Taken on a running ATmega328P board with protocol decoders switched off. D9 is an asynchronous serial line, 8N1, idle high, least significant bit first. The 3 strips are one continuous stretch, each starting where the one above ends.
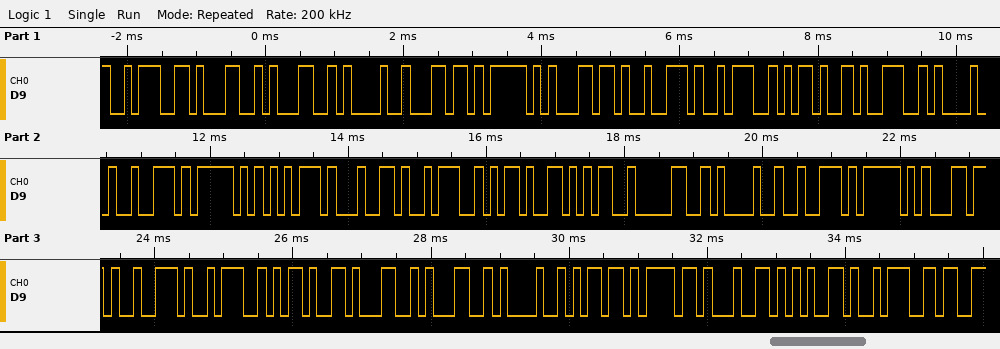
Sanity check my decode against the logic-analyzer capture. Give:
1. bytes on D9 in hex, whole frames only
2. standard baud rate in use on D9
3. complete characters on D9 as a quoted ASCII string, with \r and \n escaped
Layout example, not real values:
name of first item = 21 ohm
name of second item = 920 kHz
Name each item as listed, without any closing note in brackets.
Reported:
bytes on D9 in hex, whole frames only = 0x3A 0x31 0x31 0x21 0x6C 0x5F 0x6C 0x72 0x3A 0x2D 0x39 0x21 0x72 0x5F 0x75 0x64 0x3A 0x2D 0x35 0x30 0x21 0x72 0x5F 0x6C 0x72 0x3A 0x2D 0x31 0x31 0x21 0x6D 0x6F 0x64 0x65 0x3A
standard baud rate in use on D9 = 9600 baud
complete characters on D9 as a quoted ASCII string, with \r and \n escaped = ":11!l_lr:-9!r_ud:-50!r_lr:-11!mode:"
